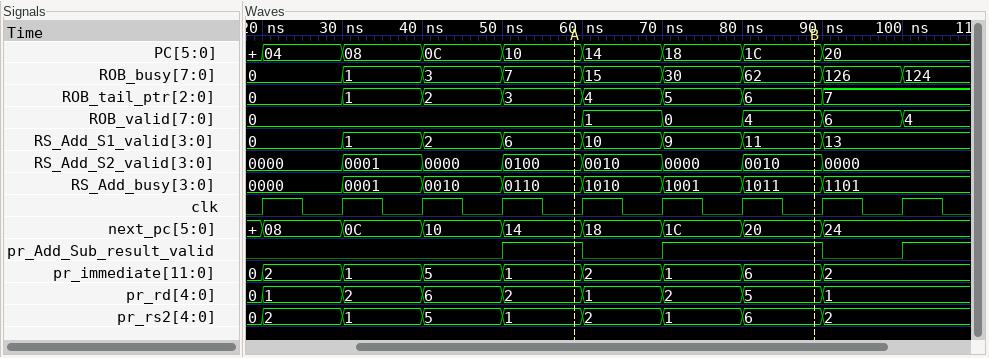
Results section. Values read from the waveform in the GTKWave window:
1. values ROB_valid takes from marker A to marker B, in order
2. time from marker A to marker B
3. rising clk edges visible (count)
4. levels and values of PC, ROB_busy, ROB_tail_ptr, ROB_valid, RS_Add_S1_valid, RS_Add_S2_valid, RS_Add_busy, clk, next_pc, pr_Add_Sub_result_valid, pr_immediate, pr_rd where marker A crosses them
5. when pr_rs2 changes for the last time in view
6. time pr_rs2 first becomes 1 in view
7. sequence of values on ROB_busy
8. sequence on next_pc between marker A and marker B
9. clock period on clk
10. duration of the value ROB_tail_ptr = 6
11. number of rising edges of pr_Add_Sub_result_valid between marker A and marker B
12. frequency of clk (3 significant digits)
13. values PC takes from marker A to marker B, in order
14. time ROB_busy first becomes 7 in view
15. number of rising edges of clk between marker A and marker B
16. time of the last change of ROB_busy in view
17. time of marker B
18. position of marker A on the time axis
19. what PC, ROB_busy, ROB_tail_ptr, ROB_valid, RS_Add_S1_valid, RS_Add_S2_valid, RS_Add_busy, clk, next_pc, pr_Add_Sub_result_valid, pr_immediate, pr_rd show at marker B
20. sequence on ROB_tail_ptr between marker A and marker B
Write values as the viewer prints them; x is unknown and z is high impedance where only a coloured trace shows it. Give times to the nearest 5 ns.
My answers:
0, 1, 0, 4
30 ns
9
PC=10, ROB_busy=7, ROB_tail_ptr=3, ROB_valid=0, RS_Add_S1_valid=6, RS_Add_S2_valid=0100, RS_Add_busy=0110, clk=0, next_pc=14, pr_Add_Sub_result_valid=1, pr_immediate=1, pr_rd=2
90 ns
30 ns
0, 1, 3, 7, 15, 30, 62, 126, 124
14, 18, 1C, 20
10 ns
10 ns
1
100 MHz
10, 14, 18, 1C
50 ns
3
100 ns
90 ns
60 ns
PC=1C, ROB_busy=62, ROB_tail_ptr=6, ROB_valid=4, RS_Add_S1_valid=11, RS_Add_S2_valid=0010, RS_Add_busy=1011, clk=0, next_pc=20, pr_Add_Sub_result_valid=1, pr_immediate=6, pr_rd=5
3, 4, 5, 6
